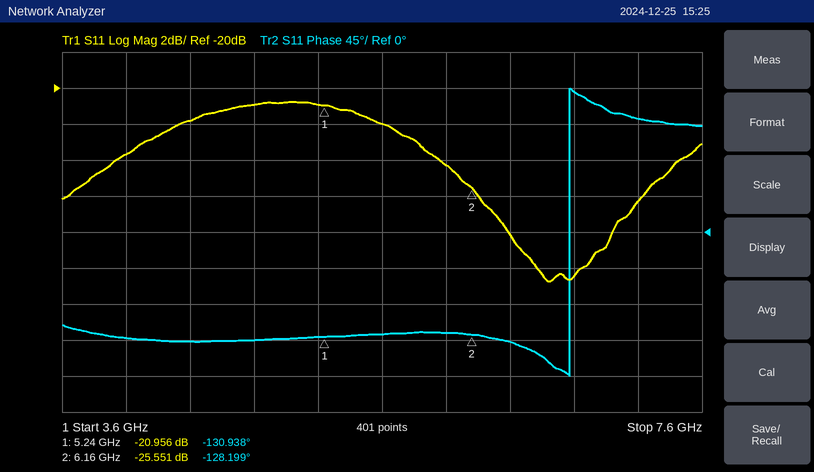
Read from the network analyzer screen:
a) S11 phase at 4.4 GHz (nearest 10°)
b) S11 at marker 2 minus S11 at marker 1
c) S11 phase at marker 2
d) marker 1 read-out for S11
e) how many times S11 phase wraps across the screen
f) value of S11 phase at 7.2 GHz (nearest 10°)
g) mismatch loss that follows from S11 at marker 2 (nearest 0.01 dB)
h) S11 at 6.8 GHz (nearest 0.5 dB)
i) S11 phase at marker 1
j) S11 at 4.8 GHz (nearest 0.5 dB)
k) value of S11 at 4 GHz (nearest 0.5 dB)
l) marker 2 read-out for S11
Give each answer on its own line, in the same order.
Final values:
-140°
-4.595 dB
-128.199°
-20.956 dB
1
140°
0.01 dB
-30.5 dB
-130.938°
-21.0 dB
-23.5 dB
-25.551 dB
